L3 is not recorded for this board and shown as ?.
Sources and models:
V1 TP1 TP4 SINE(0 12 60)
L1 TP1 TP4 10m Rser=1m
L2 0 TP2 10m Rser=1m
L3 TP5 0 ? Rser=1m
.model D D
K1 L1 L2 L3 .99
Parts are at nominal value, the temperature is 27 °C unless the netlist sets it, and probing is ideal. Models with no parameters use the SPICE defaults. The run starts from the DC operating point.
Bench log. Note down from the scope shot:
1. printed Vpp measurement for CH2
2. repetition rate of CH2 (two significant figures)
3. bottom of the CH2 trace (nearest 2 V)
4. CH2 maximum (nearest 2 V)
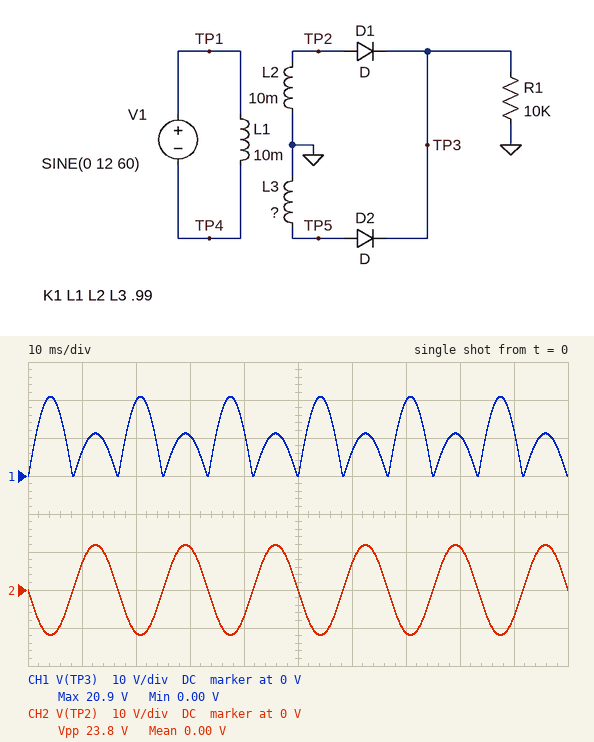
23.8 V
60 Hz
-12 V
12 V
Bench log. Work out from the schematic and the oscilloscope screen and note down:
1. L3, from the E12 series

33 mH
